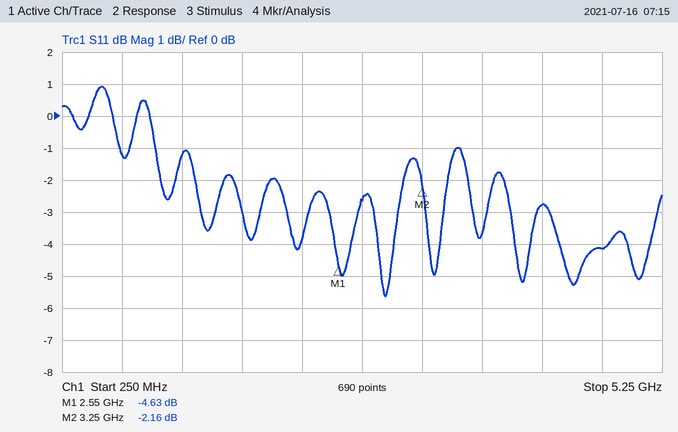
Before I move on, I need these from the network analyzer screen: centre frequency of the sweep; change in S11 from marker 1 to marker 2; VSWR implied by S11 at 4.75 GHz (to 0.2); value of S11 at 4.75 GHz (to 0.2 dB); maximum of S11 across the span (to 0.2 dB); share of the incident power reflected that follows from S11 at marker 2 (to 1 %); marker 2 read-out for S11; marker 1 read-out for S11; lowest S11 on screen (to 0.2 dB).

2.75 GHz
2.47 dB
4.2
-4.2 dB
1.0 dB
61 %
-2.16 dB
-4.63 dB
-5.6 dB
